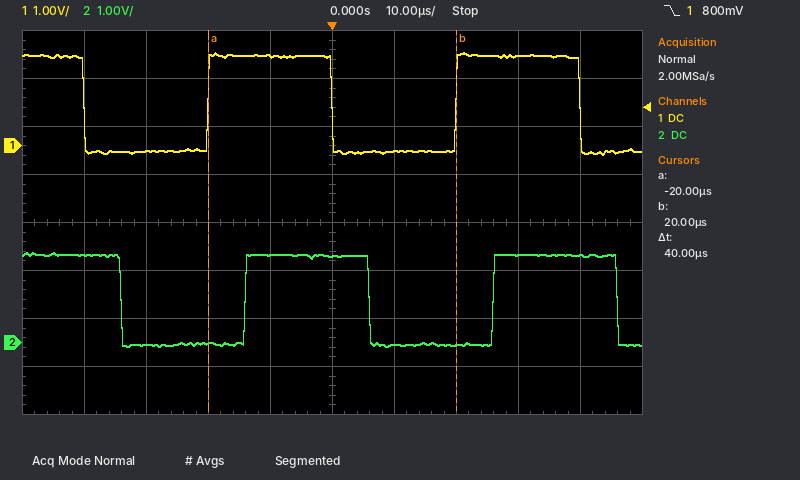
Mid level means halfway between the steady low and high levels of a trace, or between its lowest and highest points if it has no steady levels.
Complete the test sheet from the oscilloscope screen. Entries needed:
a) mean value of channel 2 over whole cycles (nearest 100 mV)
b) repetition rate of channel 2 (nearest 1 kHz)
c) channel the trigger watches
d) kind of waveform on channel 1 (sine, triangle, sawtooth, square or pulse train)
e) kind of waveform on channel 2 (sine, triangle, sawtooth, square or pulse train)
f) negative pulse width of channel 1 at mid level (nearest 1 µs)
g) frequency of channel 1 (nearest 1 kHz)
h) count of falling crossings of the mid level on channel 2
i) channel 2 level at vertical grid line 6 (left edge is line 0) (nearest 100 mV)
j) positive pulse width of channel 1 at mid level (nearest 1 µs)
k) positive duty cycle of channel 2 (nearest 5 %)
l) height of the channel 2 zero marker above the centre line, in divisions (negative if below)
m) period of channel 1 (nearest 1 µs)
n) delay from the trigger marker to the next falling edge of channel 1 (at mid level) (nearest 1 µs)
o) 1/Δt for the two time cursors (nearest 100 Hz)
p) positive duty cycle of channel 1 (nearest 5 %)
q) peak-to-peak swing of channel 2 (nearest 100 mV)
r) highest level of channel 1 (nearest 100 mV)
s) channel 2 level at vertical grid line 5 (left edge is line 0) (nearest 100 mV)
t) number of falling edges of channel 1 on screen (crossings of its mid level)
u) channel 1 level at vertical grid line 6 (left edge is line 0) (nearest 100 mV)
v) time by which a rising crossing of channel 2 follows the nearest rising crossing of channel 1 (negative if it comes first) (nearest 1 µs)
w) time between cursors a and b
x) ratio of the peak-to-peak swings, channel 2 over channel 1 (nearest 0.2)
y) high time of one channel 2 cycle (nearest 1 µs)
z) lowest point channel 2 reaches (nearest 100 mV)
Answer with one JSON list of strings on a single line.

["900 mV", "25 kHz", "channel 1", "square", "square", "20 µs", "25 kHz", "3", "0.0 V", "20 µs", "50 %", "-2.5 div", "40 µs", "40 µs", "25.0 kHz", "50 %", "2.0 V", "1.9 V", "1.8 V", "3", "-100 mV", "+6 µs", "40 µs", "1.0", "20 µs", "-100 mV"]
